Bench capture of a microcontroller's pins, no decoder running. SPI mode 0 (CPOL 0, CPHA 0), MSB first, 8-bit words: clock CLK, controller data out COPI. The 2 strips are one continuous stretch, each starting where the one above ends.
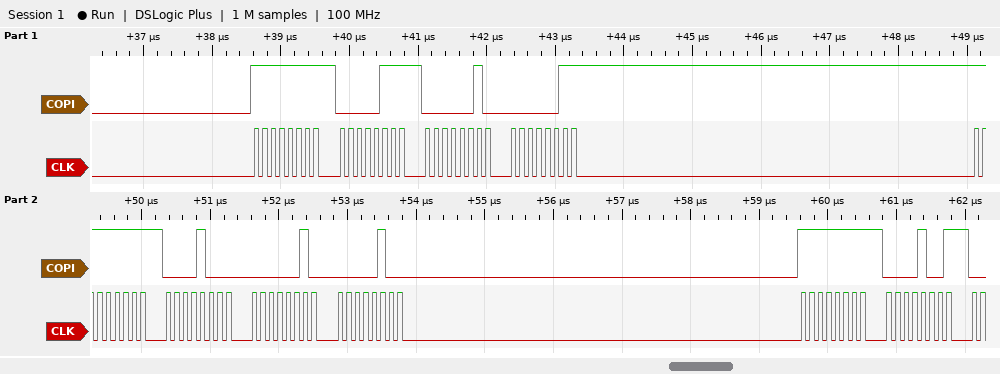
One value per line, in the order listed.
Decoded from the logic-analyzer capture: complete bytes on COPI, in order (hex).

FF 07 02 03 FF 08 02 04 FF 09
